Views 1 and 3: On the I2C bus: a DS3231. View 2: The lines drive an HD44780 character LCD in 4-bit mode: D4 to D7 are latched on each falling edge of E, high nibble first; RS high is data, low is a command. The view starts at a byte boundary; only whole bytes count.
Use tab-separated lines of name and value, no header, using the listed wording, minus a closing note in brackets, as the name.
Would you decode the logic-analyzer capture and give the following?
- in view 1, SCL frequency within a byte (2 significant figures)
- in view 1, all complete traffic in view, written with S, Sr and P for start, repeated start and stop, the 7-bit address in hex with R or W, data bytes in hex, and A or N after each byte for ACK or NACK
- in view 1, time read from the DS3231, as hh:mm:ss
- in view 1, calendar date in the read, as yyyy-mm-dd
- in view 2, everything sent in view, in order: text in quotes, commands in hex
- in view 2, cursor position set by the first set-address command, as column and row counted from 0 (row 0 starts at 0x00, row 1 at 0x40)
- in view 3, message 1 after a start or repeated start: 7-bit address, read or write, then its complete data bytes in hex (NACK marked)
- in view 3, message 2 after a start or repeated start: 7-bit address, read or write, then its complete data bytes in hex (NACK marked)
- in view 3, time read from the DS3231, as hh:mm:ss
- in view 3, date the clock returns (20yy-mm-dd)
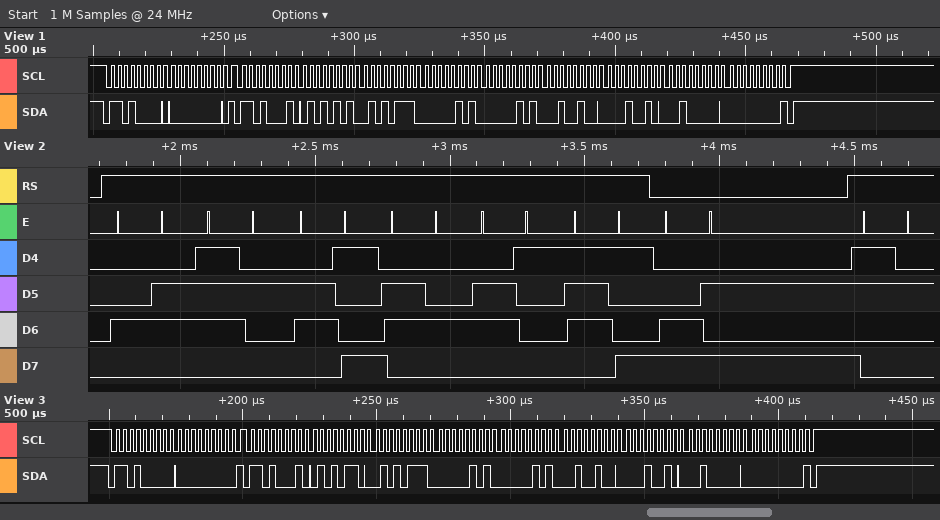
in view 1, SCL frequency within a byte	400 kHz
in view 1, all complete traffic in view, written with S, Sr and P for start, repeated start and stop, the 7-bit address in hex with R or W, data bytes in hex, and A or N after each byte for ACK or NACK	S 68W A 00 A Sr 68R A 55 A 57 A 05 A 05 A 24 A 12 A 20 A 00 N P
in view 1, time read from the DS3231, as hh:mm:ss	05:57:55
in view 1, calendar date in the read, as yyyy-mm-dd	2020-12-24
in view 2, everything sent in view, in order: text in quotes, commands in hex	"Friday" 0xCA "2"
in view 2, cursor position set by the first set-address command, as column and row counted from 0	column 10, row 1
in view 3, message 1 after a start or repeated start: 7-bit address, read or write, then its complete data bytes in hex	0x68 write: 00
in view 3, message 2 after a start or repeated start: 7-bit address, read or write, then its complete data bytes in hex	0x68 read: 56 57 05 05 24 12 20 00 NACK
in view 3, time read from the DS3231, as hh:mm:ss	05:57:56
in view 3, date the clock returns	2020-12-24
